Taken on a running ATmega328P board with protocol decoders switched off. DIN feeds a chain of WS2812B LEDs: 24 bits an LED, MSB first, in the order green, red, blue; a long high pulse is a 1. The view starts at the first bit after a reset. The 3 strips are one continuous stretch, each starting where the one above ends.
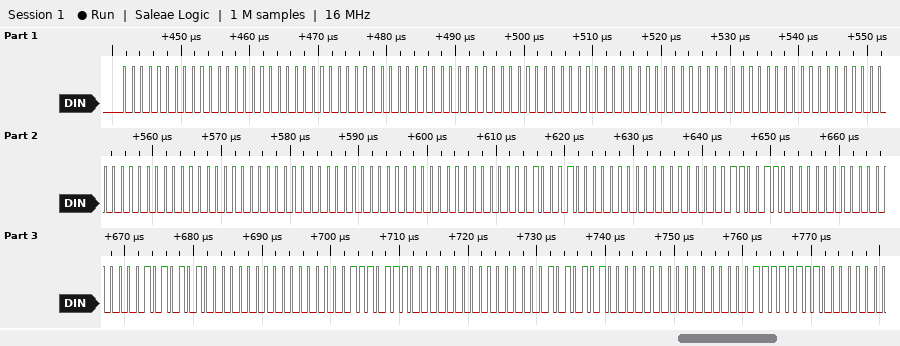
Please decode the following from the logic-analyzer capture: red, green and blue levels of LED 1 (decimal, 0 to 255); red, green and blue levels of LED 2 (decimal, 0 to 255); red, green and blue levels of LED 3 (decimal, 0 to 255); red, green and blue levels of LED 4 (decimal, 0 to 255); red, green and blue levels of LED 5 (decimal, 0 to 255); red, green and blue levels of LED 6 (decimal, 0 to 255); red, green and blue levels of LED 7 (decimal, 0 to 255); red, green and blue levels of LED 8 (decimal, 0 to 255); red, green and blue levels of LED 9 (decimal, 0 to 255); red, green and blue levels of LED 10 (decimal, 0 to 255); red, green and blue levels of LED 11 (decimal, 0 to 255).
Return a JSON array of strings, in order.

["0, 0, 0", "0, 0, 0", "0, 0, 0", "0, 0, 0", "0, 0, 0", "0, 0, 17", "0, 0, 51", "0, 0, 85", "0, 0, 119", "0, 0, 170", "0, 0, 255"]
